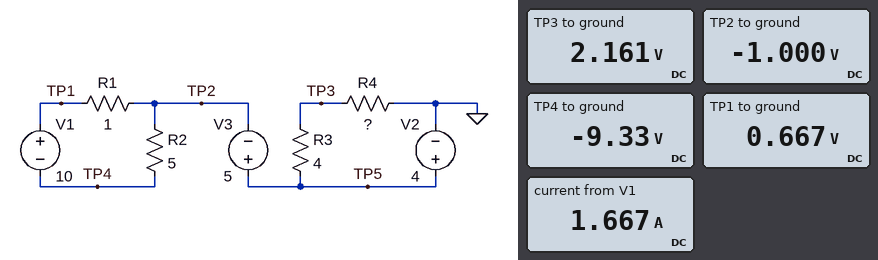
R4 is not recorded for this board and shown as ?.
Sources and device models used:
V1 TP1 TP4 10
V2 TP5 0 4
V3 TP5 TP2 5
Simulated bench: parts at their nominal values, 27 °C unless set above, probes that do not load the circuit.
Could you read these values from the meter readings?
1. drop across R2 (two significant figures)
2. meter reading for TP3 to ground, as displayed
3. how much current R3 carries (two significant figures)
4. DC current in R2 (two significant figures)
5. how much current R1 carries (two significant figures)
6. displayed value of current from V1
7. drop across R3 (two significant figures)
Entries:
8.3 V
2.161 V
460 mA
1.7 A
1.7 A
1.667 A
1.8 V
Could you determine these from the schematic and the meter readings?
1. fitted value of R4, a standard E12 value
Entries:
4.7 Ω
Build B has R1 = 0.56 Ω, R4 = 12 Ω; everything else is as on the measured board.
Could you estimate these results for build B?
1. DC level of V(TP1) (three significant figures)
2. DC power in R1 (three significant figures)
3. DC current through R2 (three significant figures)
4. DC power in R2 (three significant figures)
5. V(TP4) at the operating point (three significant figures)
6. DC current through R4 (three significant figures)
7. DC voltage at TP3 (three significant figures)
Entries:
7.19 mV
1.81 W
1.80 A
16.2 W
-9.99 V
250 mA
3.00 V
